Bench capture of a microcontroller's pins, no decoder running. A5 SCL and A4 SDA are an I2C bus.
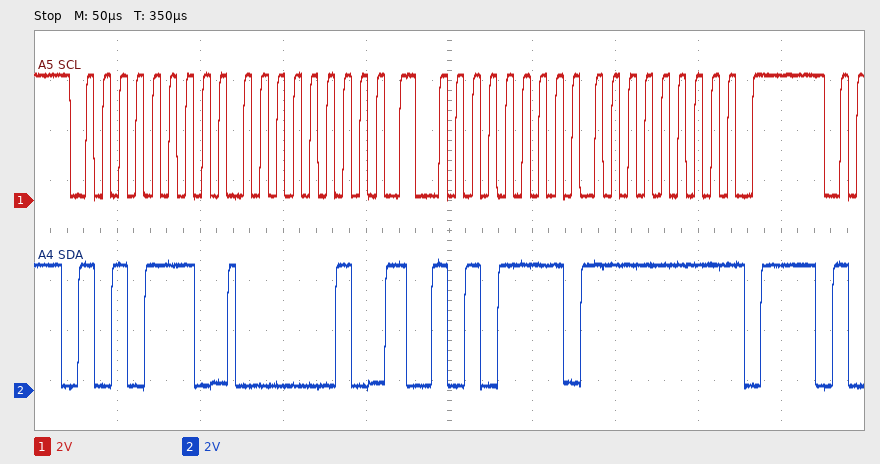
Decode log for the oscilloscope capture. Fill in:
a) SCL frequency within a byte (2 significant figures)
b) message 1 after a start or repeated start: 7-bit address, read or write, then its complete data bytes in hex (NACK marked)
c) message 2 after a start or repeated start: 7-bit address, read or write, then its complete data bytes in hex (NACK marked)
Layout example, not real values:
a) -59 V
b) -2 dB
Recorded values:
a) 100 kHz
b) 0x57 write: 02
c) 0x57 read: FF NACK
